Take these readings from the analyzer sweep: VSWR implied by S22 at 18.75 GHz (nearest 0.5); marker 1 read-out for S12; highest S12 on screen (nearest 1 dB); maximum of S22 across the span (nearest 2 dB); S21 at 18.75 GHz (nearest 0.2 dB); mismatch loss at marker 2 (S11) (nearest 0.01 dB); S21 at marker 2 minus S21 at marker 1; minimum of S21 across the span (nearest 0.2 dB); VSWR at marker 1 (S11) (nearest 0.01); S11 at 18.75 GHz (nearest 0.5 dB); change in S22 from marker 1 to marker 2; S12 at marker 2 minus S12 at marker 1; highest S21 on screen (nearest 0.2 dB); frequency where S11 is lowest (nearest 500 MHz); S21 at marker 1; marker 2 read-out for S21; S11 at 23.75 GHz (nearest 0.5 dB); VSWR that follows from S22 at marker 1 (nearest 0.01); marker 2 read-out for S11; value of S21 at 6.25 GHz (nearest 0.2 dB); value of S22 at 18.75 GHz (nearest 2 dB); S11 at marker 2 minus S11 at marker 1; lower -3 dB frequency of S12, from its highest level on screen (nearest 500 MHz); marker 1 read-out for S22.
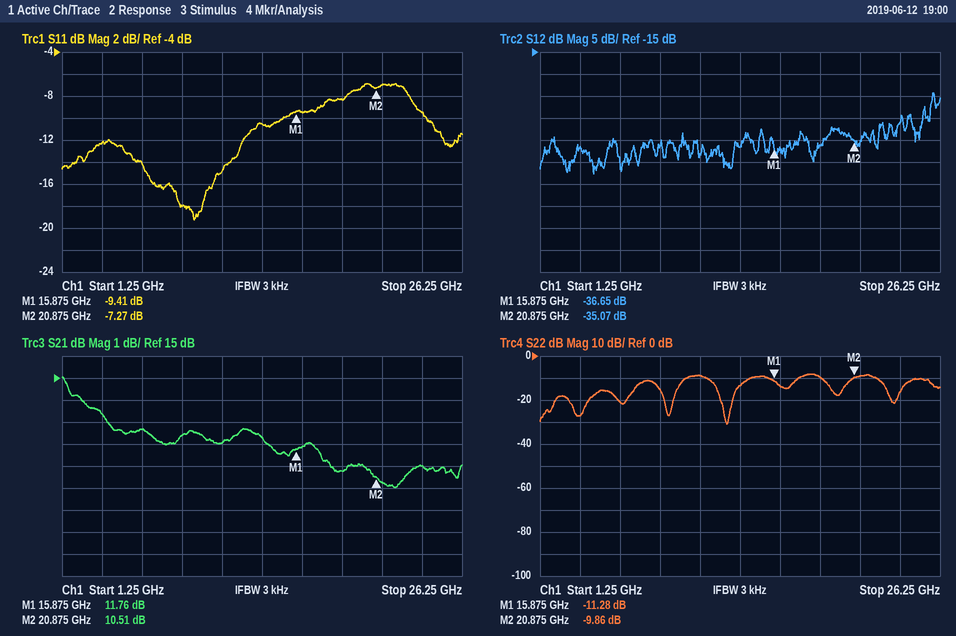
2.0
-36.65 dB
-24 dB
-8 dB
10.8 dB
0.90 dB
-1.25 dB
10.0 dB
2.02
-8.5 dB
1.42 dB
1.58 dB
15.0 dB
9.5 GHz
11.76 dB
10.51 dB
-9.5 dB
1.75
-7.27 dB
12.6 dB
-10 dB
2.14 dB
25.5 GHz
-11.28 dB
